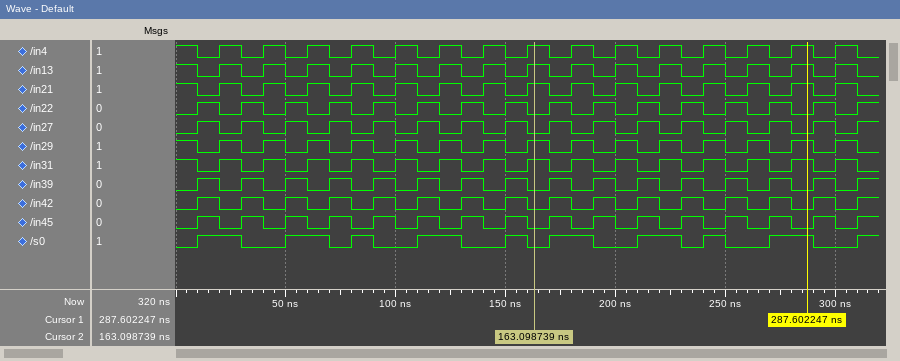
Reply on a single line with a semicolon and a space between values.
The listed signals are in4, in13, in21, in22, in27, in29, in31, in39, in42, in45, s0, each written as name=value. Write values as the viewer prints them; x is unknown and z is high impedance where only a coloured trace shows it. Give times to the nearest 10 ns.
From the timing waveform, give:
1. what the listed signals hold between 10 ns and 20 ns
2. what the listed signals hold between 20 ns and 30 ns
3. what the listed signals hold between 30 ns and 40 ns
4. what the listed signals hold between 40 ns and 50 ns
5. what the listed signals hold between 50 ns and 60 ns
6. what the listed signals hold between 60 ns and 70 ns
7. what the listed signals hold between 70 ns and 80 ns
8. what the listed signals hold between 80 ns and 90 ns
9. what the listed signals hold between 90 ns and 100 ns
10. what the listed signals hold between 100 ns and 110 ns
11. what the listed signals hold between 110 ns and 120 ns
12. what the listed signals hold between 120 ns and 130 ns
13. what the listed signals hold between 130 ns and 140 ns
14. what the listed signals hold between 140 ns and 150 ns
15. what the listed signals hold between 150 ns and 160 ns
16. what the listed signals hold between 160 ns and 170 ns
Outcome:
in4=0, in13=0, in21=0, in22=1, in27=1, in29=0, in31=0, in39=1, in42=1, in45=1, s0=1; in4=1, in13=1, in21=1, in22=0, in27=0, in29=1, in31=1, in39=0, in42=0, in45=0, s0=1; in4=0, in13=0, in21=0, in22=1, in27=1, in29=0, in31=0, in39=1, in42=1, in45=1, s0=0; in4=1, in13=1, in21=1, in22=0, in27=0, in29=1, in31=1, in39=0, in42=0, in45=0, s0=0; in4=0, in13=0, in21=0, in22=1, in27=1, in29=0, in31=0, in39=1, in42=1, in45=1, s0=1; in4=1, in13=1, in21=1, in22=0, in27=0, in29=1, in31=1, in39=0, in42=0, in45=0, s0=1; in4=0, in13=0, in21=0, in22=1, in27=1, in29=0, in31=0, in39=1, in42=1, in45=1, s0=0; in4=1, in13=1, in21=1, in22=0, in27=0, in29=1, in31=1, in39=0, in42=0, in45=0, s0=1; in4=0, in13=0, in21=0, in22=1, in27=1, in29=0, in31=0, in39=1, in42=1, in45=1, s0=0; in4=1, in13=1, in21=1, in22=0, in27=0, in29=1, in31=1, in39=0, in42=0, in45=0, s0=0; in4=0, in13=0, in21=0, in22=1, in27=1, in29=0, in31=0, in39=1, in42=1, in45=1, s0=1; in4=1, in13=1, in21=1, in22=0, in27=0, in29=1, in31=1, in39=0, in42=0, in45=0, s0=1; in4=0, in13=0, in21=0, in22=1, in27=1, in29=0, in31=0, in39=1, in42=1, in45=1, s0=0; in4=1, in13=1, in21=1, in22=0, in27=0, in29=1, in31=1, in39=0, in42=0, in45=0, s0=0; in4=0, in13=0, in21=0, in22=1, in27=1, in29=0, in31=0, in39=1, in42=1, in45=1, s0=1; in4=1, in13=1, in21=1, in22=0, in27=0, in29=1, in31=1, in39=0, in42=0, in45=0, s0=0
